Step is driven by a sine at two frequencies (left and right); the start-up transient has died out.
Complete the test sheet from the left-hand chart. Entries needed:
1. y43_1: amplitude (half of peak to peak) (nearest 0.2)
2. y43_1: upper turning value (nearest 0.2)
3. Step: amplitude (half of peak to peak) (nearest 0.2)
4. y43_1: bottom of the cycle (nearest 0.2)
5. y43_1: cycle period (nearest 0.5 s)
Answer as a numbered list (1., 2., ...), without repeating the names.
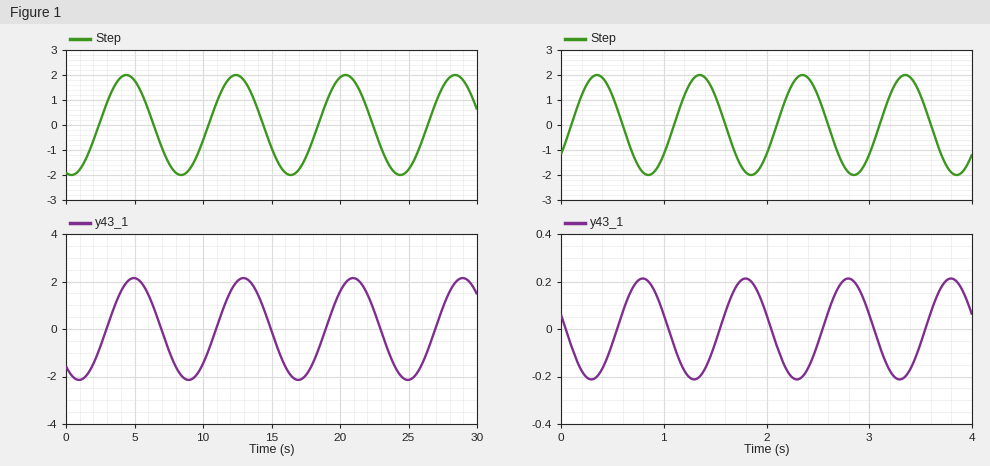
1. 2.2
2. 2.2
3. 2.0
4. -2.2
5. 8.0 s
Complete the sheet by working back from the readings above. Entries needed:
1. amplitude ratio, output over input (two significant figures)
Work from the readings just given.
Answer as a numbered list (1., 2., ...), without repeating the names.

1. 1.1
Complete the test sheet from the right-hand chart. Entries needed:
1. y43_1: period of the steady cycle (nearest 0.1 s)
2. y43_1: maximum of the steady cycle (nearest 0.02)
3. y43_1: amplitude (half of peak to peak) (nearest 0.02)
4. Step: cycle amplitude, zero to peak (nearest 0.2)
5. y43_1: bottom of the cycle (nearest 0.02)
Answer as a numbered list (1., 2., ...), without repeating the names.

1. 1.0 s
2. 0.22
3. 0.22
4. 2.0
5. -0.22
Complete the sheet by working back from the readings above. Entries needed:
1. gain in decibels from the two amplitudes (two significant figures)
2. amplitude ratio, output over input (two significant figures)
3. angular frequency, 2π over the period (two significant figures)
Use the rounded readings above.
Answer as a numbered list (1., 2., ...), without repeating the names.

1. -19 dB
2. 0.11
3. 6.3 rad/s
